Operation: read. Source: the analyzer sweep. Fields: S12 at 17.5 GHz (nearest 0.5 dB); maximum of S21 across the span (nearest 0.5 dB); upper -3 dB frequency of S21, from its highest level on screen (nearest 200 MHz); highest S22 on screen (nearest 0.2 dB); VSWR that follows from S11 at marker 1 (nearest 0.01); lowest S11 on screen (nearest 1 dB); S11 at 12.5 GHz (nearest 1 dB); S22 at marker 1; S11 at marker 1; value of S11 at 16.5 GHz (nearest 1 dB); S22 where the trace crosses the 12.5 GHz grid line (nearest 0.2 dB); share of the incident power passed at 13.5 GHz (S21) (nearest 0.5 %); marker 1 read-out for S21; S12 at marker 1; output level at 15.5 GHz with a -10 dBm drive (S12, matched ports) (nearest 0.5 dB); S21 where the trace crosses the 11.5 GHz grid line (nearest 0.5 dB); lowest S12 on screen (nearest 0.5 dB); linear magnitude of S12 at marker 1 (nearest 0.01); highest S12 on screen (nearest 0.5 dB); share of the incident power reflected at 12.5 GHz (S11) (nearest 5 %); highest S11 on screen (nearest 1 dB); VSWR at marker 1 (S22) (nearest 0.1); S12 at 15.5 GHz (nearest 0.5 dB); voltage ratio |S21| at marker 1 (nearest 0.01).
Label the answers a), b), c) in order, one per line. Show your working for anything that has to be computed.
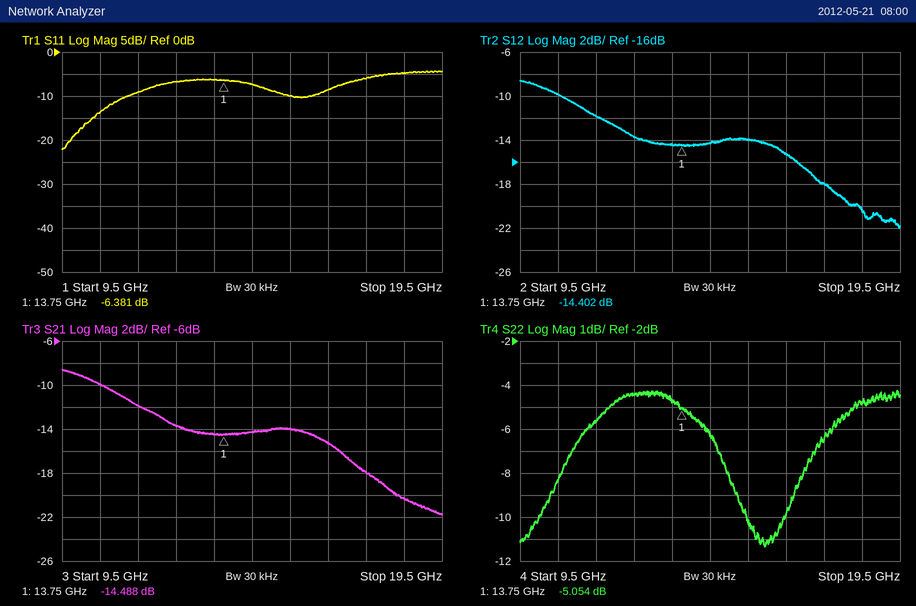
a) -18.0 dB
b) -8.5 dB
c) 11.4 GHz
d) -4.2 dB
e) (1 + 0.4797)/(1 − 0.4797) ≈ 2.84
f) -22 dB
g) -7 dB
h) -5.054 dB
i) -6.381 dB
j) -9 dB
k) -4.4 dB
l) 10^(-14.5/10) ≈ 3.5 %
m) -14.488 dB
n) -14.402 dB
o) -10 dBm + (-14.0 dB) = -24.0 dBm
p) -12.0 dB
q) -22.0 dB
r) 10^(-14.402/20) ≈ 0.19
s) -8.5 dB
t) 10^(-7/10) ≈ 20 %
u) -4 dB
v) (1 + 0.5589)/(1 − 0.5589) ≈ 3.5
w) -14.0 dB
x) 10^(-14.488/20) ≈ 0.19
